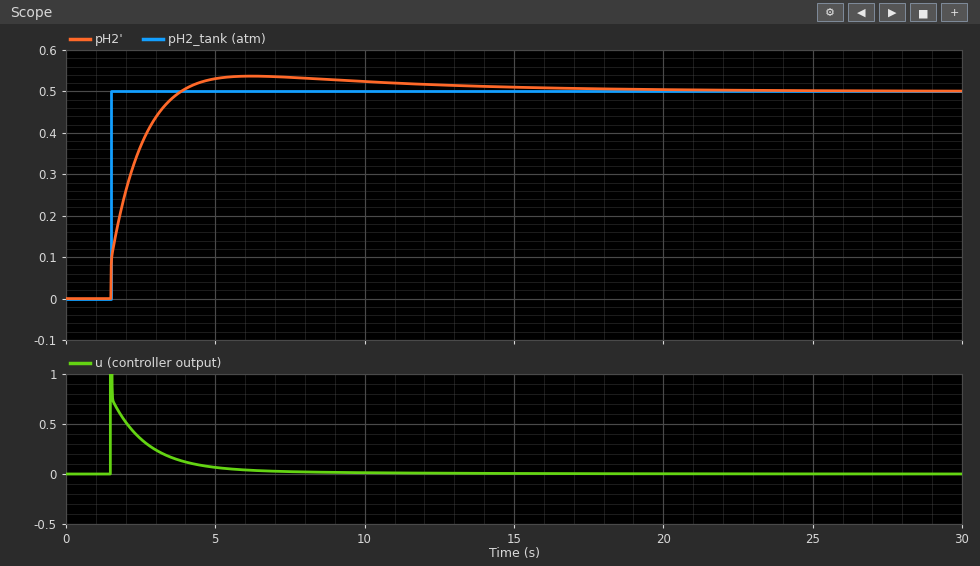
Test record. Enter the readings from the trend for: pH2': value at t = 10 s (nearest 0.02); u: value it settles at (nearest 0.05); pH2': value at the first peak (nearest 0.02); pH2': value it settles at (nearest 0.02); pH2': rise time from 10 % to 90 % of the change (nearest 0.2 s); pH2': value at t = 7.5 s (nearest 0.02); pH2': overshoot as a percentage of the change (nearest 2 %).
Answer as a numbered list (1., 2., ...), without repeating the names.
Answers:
1. 0.52
2. 0.00
3. 0.54
4. 0.50
5. 1.6 s
6. 0.54
7. 8 %
